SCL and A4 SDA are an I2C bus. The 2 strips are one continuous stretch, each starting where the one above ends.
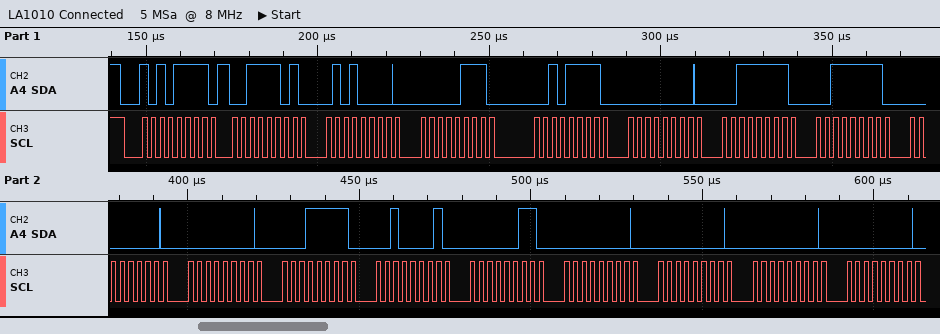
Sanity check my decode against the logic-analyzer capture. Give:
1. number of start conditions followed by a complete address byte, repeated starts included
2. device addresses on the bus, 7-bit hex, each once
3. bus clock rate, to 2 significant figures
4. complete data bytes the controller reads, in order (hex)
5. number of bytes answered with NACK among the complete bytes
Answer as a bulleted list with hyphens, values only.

- 1
- 0x57
- 400 kHz
- 3D 50 07 2F 00 3F 3F 00 00 1F 21 03 00 00 00 00
- 0
